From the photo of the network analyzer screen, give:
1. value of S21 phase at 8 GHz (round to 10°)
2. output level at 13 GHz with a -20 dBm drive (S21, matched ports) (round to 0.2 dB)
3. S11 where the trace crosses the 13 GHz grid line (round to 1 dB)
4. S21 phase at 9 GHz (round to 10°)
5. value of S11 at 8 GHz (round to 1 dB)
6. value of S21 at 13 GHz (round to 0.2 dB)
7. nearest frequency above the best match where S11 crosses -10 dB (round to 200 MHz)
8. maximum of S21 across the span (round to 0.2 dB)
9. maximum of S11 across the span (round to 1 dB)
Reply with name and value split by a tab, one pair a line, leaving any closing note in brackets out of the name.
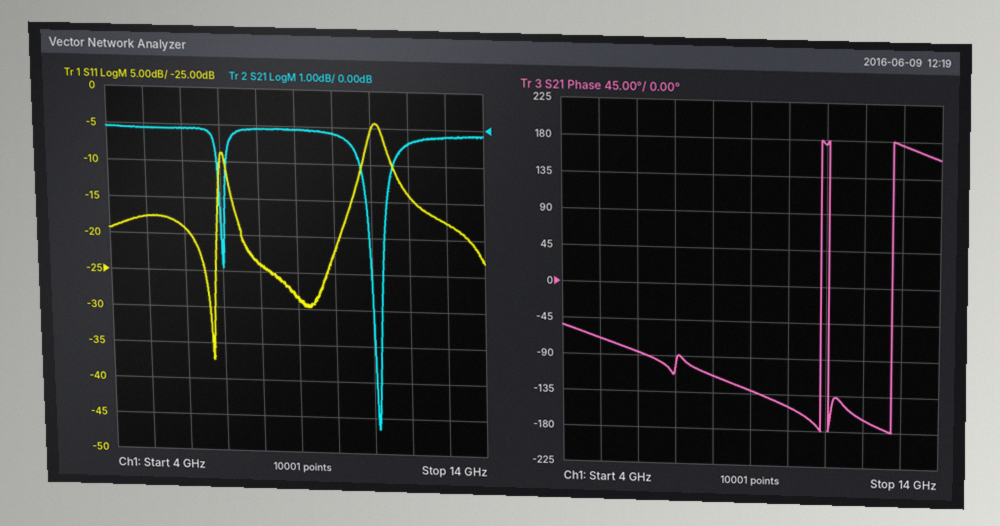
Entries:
value of S21 phase at 8 GHz	-110°
output level at 13 GHz with a -20 dBm drive (S21, matched ports)	-20.2 dBm
S11 where the trace crosses the 13 GHz grid line	-18 dB
S21 phase at 9 GHz	-130°
value of S11 at 8 GHz	-24 dB
value of S21 at 13 GHz	-0.2 dB
nearest frequency above the best match where S11 crosses -10 dB	7.0 GHz
maximum of S21 across the span	0.0 dB
maximum of S11 across the span	-4 dB
